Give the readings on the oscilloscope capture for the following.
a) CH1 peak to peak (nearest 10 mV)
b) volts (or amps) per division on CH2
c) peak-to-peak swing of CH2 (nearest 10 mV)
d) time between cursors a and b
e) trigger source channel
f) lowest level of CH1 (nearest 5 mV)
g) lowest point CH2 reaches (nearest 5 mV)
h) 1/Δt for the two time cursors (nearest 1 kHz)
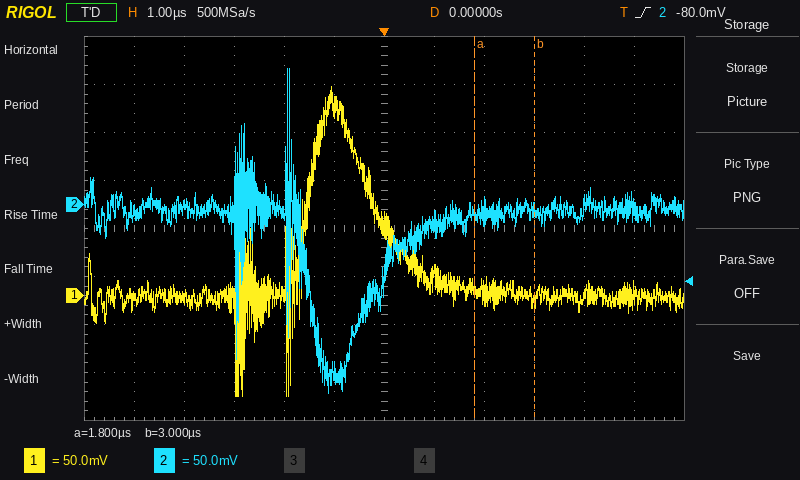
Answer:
320 mV
50 mV
340 mV
1.2 µs
CH2
-105 mV
-195 mV
833 kHz
